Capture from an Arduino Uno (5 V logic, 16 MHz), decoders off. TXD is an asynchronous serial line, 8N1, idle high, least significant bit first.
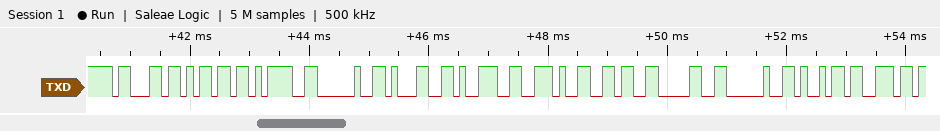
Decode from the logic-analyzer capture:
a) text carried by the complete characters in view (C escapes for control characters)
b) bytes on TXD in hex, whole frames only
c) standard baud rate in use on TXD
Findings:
"cm= 19.60 in"
63 6D 3D 20 31 39 2E 36 30 20 69 6E
9600 baud
